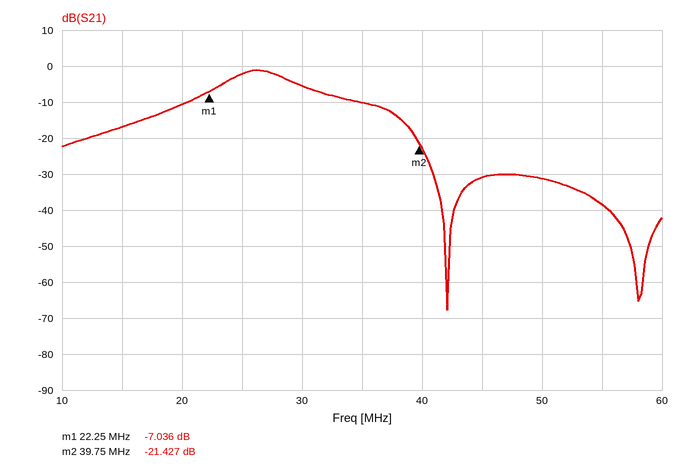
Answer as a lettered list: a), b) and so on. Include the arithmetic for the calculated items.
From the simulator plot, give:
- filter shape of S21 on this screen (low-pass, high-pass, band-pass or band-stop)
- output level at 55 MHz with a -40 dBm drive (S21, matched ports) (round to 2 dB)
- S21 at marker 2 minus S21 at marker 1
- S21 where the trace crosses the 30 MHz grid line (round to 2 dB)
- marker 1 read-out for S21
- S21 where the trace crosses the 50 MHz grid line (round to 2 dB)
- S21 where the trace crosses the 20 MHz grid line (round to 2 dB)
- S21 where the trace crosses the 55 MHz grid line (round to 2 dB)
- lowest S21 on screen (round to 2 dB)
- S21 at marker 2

a) band-pass
b) -40 dBm + (-38 dB) = -78 dBm
c) -21.427 − (-7.036) = -14.391 dB
d) -6 dB
e) -7.036 dB
f) -32 dB
g) -10 dB
h) -38 dB
i) -68 dB
j) -21.427 dB
